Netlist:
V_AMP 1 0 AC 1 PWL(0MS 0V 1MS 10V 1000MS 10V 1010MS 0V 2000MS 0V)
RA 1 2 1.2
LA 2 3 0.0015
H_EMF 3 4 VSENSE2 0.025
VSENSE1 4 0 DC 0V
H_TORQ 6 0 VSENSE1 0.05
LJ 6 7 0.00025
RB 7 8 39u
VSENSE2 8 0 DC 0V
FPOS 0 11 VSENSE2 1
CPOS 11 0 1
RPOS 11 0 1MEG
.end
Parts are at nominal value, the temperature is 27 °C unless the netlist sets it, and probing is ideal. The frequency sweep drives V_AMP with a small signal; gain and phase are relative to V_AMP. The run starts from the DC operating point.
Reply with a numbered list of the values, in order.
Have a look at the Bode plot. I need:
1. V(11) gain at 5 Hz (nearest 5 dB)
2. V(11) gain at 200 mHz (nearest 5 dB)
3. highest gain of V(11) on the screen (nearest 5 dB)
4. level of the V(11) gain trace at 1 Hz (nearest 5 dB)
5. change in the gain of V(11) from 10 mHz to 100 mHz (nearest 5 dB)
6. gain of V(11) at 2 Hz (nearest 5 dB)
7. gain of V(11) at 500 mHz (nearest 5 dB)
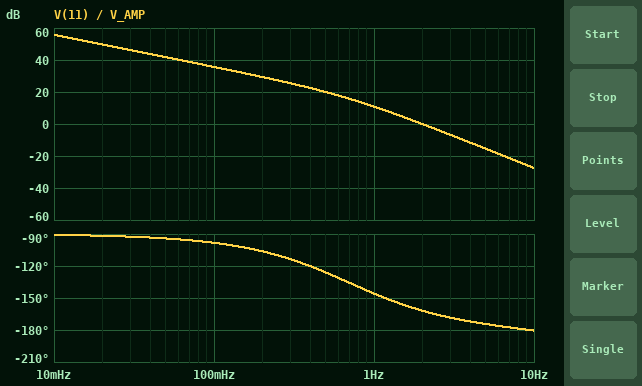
1. -15 dB
2. 30 dB
3. 55 dB
4. 10 dB
5. -20 dB
6. 0 dB
7. 20 dB
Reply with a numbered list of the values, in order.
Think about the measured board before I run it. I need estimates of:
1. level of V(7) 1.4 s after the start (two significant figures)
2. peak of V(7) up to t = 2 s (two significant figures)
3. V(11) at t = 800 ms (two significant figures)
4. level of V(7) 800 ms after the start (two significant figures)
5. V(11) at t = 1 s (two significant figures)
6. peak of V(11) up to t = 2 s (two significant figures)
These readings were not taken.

1. 2.7 mV
2. 15 mV
3. 220 V
4. 15 mV
5. 300 V
6. 390 V
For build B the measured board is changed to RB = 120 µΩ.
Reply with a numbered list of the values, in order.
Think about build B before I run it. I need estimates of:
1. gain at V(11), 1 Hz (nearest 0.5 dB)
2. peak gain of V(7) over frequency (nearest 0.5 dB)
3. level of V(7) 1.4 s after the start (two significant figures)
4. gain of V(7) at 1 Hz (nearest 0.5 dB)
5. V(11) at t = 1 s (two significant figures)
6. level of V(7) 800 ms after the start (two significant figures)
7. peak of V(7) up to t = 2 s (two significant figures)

1. 10.5 dB
2. -47.5 dB
3. 6.8 mV
4. -52.0 dB
5. 280 V
6. 42 mV
7. 43 mV
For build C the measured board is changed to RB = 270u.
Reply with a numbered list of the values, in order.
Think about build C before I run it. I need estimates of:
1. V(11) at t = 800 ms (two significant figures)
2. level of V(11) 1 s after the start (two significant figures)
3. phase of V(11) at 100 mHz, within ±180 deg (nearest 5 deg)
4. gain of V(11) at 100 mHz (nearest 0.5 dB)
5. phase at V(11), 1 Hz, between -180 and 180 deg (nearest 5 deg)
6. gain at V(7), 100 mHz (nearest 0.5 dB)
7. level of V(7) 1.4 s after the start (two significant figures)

1. 190 V
2. 260 V
3. -95 deg
4. 34.0 dB
5. -140 deg
6. -41.5 dB
7. 11 mV
